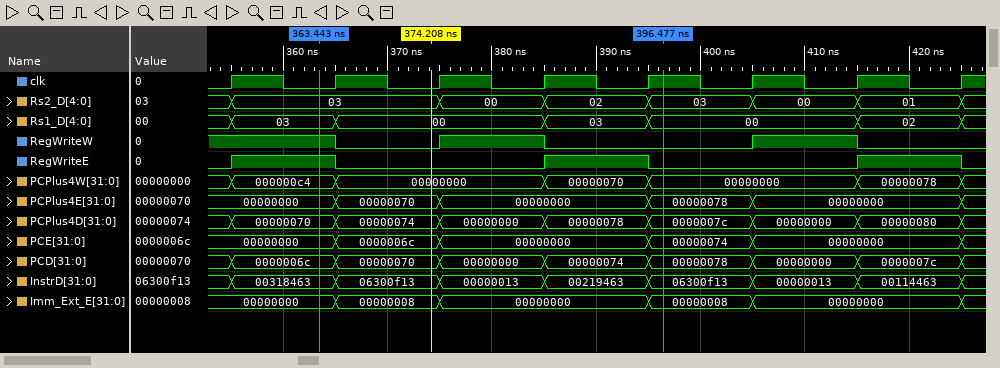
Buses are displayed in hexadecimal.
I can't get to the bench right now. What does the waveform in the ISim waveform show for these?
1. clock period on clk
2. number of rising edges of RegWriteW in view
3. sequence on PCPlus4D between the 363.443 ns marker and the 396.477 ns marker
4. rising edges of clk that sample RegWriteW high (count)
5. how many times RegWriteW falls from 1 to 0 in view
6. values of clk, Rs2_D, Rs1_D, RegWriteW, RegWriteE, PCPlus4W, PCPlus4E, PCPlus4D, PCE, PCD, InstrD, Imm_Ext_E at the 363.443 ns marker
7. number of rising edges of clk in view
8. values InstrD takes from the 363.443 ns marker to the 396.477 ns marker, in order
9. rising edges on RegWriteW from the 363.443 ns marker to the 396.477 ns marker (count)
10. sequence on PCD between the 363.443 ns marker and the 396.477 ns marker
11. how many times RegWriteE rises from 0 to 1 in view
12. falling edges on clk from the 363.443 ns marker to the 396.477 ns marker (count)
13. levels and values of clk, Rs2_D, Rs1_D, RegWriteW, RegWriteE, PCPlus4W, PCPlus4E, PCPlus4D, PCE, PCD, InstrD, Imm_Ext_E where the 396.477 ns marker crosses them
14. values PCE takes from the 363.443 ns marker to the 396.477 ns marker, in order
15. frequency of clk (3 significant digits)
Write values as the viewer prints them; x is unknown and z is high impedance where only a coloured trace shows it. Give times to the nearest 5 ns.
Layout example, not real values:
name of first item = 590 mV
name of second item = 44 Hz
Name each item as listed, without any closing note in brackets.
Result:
clock period on clk = 10 ns
number of rising edges of RegWriteW in view = 2
sequence on PCPlus4D between the 363.443 ns marker and the 396.477 ns marker = 00000070, 00000074, 00000000, 00000078, 0000007c
rising edges of clk that sample RegWriteW high = 4
how many times RegWriteW falls from 1 to 0 in view = 3
values of clk, Rs2_D, Rs1_D, RegWriteW, RegWriteE, PCPlus4W, PCPlus4E, PCPlus4D, PCE, PCD, InstrD, Imm_Ext_E at the 363.443 ns marker = clk=0, Rs2_D=03, Rs1_D=03, RegWriteW=1, RegWriteE=1, PCPlus4W=000000c4, PCPlus4E=00000000, PCPlus4D=00000070, PCE=00000000, PCD=0000006c, InstrD=00318463, Imm_Ext_E=00000000
number of rising edges of clk in view = 8
values InstrD takes from the 363.443 ns marker to the 396.477 ns marker, in order = 00318463, 06300f13, 00000013, 00219463, 06300f13
rising edges on RegWriteW from the 363.443 ns marker to the 396.477 ns marker = 1
sequence on PCD between the 363.443 ns marker and the 396.477 ns marker = 0000006c, 00000070, 00000000, 00000074, 00000078
how many times RegWriteE rises from 0 to 1 in view = 3
falling edges on clk from the 363.443 ns marker to the 396.477 ns marker = 3
levels and values of clk, Rs2_D, Rs1_D, RegWriteW, RegWriteE, PCPlus4W, PCPlus4E, PCPlus4D, PCE, PCD, InstrD, Imm_Ext_E where the 396.477 ns marker crosses them = clk=1, Rs2_D=03, Rs1_D=00, RegWriteW=0, RegWriteE=0, PCPlus4W=00000000, PCPlus4E=00000078, PCPlus4D=0000007c, PCE=00000074, PCD=00000078, InstrD=06300f13, Imm_Ext_E=00000008
values PCE takes from the 363.443 ns marker to the 396.477 ns marker, in order = 00000000, 0000006c, 00000000, 00000074
frequency of clk = 100 MHz
